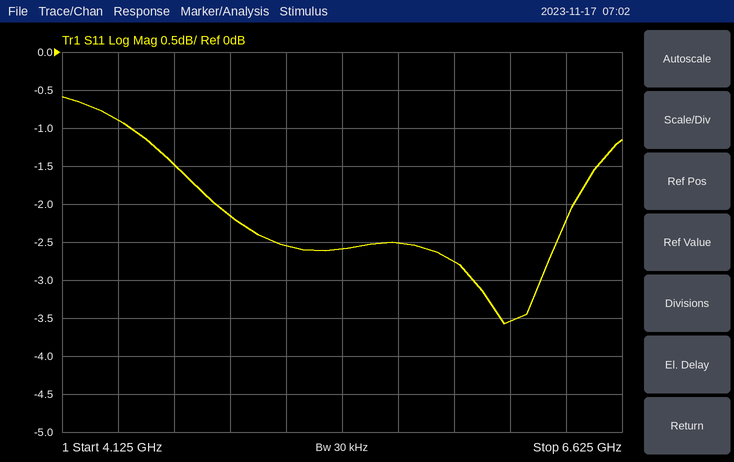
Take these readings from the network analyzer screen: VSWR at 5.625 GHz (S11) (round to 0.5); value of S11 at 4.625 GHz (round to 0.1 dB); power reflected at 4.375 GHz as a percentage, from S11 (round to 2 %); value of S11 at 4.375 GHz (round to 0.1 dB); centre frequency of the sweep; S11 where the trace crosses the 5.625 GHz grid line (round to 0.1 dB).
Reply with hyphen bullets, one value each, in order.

- 7.0
- -1.5 dB
- 82 %
- -0.9 dB
- 5.375 GHz
- -2.5 dB
